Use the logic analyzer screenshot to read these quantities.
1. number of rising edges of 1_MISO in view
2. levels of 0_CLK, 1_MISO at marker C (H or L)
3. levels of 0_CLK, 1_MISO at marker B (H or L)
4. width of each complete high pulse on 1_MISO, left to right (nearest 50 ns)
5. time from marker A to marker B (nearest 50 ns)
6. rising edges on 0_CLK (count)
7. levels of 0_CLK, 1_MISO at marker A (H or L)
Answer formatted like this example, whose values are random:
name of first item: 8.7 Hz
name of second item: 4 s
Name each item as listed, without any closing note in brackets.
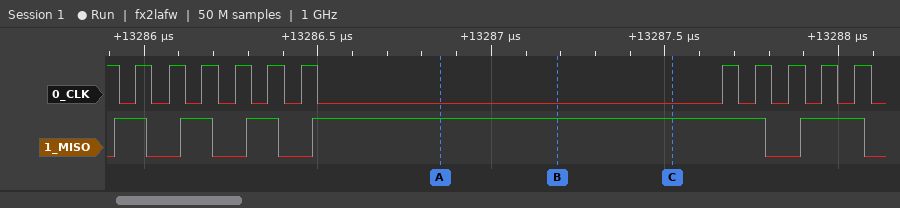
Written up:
number of rising edges of 1_MISO in view: 5
levels of 0_CLK, 1_MISO at marker C: 0_CLK=L, 1_MISO=H
levels of 0_CLK, 1_MISO at marker B: 0_CLK=L, 1_MISO=H
width of each complete high pulse on 1_MISO, left to right: 100 ns, 100 ns, 100 ns, 1300 ns, 200 ns
time from marker A to marker B: 350 ns
rising edges on 0_CLK: 11
levels of 0_CLK, 1_MISO at marker A: 0_CLK=L, 1_MISO=H
